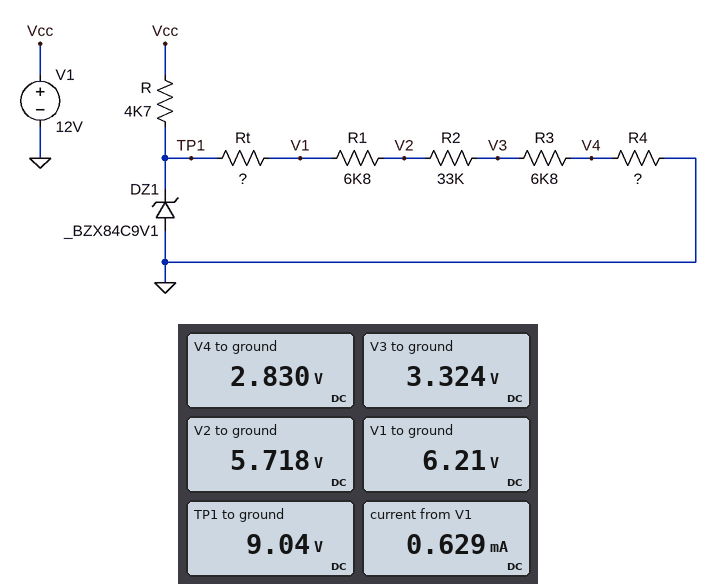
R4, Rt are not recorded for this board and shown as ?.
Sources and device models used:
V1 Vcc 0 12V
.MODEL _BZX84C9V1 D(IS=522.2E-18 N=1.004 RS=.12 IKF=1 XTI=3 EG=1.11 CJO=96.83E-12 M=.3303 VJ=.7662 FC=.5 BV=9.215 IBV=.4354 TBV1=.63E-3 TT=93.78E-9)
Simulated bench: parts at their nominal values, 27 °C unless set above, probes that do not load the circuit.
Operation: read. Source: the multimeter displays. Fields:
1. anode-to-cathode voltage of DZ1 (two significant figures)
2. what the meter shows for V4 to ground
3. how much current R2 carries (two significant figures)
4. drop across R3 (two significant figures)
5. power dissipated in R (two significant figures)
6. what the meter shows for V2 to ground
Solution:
-9.0 V
2.830 V
73 µA
490 mV
1.9 mW
5.718 V
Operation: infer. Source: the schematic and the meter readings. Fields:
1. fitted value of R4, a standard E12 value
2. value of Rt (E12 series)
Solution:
39 kΩ
39 kΩ
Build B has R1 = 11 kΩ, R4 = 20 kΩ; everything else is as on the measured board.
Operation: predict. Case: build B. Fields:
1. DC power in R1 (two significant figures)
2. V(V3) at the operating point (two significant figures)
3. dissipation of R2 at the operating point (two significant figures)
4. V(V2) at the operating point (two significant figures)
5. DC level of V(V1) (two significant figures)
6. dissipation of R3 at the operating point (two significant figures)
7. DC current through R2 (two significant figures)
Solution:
75 µW
2.2 V
220 µW
4.9 V
5.8 V
46 µW
82 µA
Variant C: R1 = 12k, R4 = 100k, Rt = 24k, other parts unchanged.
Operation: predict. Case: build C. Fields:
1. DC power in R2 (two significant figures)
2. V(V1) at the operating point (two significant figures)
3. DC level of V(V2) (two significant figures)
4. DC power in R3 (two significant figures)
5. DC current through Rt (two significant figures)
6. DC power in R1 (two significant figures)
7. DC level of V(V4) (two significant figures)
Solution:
87 µW
7.8 V
7.2 V
18 µW
51 µA
32 µW
5.1 V
